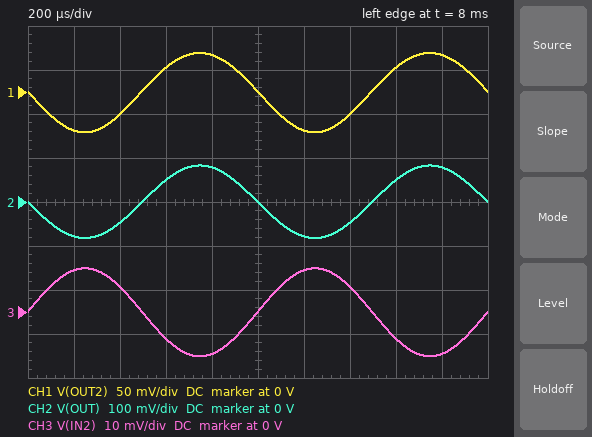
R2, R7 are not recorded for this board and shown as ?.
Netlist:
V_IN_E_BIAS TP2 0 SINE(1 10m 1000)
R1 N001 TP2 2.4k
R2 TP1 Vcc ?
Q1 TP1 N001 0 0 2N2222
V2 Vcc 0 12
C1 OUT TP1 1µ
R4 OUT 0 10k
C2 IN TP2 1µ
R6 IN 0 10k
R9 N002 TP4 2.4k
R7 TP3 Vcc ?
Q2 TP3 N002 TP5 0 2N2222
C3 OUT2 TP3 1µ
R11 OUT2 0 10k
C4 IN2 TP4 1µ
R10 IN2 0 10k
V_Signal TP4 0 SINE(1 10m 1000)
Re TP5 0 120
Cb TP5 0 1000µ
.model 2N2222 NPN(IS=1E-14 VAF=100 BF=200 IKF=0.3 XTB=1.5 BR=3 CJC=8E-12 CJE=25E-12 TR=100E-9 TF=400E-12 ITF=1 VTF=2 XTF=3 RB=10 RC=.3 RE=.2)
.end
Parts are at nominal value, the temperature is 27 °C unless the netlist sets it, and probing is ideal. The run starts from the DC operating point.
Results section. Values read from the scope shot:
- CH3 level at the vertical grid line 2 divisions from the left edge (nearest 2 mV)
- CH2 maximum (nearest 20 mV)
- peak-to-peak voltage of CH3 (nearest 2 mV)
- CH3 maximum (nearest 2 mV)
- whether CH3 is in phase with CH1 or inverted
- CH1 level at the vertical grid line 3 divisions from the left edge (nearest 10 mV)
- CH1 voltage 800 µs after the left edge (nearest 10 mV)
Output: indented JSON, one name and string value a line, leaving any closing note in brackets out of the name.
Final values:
{
  "CH3 level at the vertical grid line 2 divisions from the left edge": "6 mV",
  "CH2 maximum": "80 mV",
  "peak-to-peak voltage of CH3": "20 mV",
  "CH3 maximum": "10 mV",
  "whether CH3 is in phase with CH1 or inverted": "inverted",
  "CH1 level at the vertical grid line 3 divisions from the left edge": "30 mV",
  "CH1 voltage 800 µs after the left edge": "40 mV"
}
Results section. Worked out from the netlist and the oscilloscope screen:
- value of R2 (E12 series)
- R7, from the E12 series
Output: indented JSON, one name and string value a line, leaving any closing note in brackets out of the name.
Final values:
{
  "value of R2": "120 Ω",
  "R7, from the E12 series": "100 Ω"
}
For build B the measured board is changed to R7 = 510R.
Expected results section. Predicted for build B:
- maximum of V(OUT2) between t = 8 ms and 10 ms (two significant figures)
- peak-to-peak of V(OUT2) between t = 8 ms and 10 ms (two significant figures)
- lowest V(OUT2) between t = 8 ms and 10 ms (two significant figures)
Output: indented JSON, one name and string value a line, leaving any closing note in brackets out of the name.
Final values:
{
  "maximum of V(OUT2) between t = 8 ms and 10 ms": "210 mV",
  "peak-to-peak of V(OUT2) between t = 8 ms and 10 ms": "440 mV",
  "lowest V(OUT2) between t = 8 ms and 10 ms": "-220 mV"
}
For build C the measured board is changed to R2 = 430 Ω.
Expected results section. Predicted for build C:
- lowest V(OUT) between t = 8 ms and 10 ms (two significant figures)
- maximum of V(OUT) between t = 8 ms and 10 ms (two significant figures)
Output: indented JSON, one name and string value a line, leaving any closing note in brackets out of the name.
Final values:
{
  "lowest V(OUT) between t = 8 ms and 10 ms": "-250 mV",
  "maximum of V(OUT) between t = 8 ms and 10 ms": "260 mV"
}
